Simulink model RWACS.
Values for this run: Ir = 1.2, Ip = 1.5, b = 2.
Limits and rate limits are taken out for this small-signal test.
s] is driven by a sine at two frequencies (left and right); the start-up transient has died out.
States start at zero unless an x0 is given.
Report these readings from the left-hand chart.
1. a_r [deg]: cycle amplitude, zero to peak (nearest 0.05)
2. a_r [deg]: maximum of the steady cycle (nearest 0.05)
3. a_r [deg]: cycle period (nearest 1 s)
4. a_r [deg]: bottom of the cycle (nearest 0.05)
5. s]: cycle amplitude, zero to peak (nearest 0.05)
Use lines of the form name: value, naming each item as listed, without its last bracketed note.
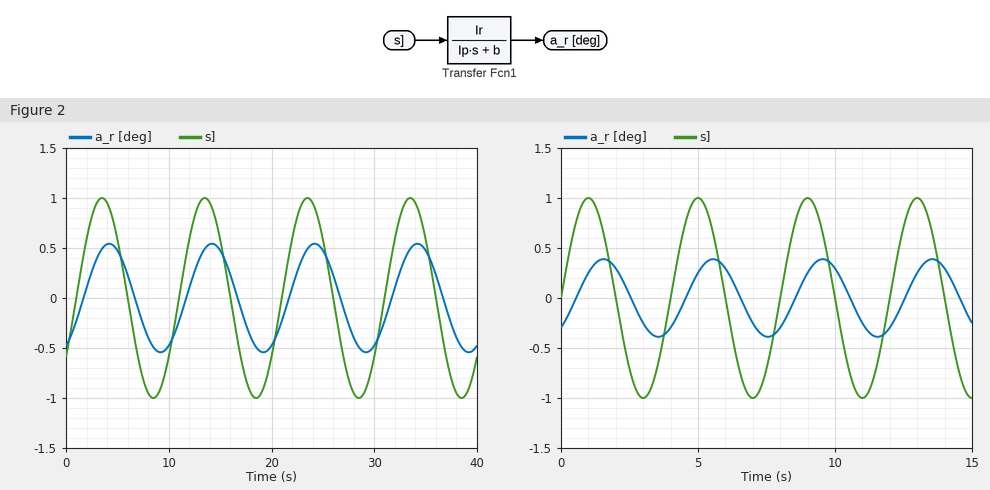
a_r [deg]: cycle amplitude, zero to peak: 0.55
a_r [deg]: maximum of the steady cycle: 0.55
a_r [deg]: cycle period: 10 s
a_r [deg]: bottom of the cycle: -0.55
s]: cycle amplitude, zero to peak: 1.00
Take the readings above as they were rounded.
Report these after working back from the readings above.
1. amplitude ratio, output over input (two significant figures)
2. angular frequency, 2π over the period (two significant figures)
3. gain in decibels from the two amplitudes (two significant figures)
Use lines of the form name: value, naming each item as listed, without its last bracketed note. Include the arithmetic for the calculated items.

amplitude ratio, output over input: 0.55 / 1 = 0.55
angular frequency, 2π over the period: 2π / 10 = 0.63 rad/s
gain in decibels from the two amplitudes: 20 log10(0.55 / 1) = -5.2 dB
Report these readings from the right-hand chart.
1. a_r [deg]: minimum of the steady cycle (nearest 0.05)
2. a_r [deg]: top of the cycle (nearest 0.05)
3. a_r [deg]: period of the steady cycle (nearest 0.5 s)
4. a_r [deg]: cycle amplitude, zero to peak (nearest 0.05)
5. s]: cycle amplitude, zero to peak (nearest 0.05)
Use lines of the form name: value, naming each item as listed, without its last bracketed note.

a_r [deg]: minimum of the steady cycle: -0.40
a_r [deg]: top of the cycle: 0.40
a_r [deg]: period of the steady cycle: 4.0 s
a_r [deg]: cycle amplitude, zero to peak: 0.40
s]: cycle amplitude, zero to peak: 1.00
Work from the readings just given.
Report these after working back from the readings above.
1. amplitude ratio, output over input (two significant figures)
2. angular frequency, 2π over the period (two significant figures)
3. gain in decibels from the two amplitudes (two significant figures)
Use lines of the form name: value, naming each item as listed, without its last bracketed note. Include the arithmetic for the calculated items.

amplitude ratio, output over input: 0.4 / 1 = 0.40
angular frequency, 2π over the period: 2π / 4 = 1.6 rad/s
gain in decibels from the two amplitudes: 20 log10(0.4 / 1) = -8.0 dB
